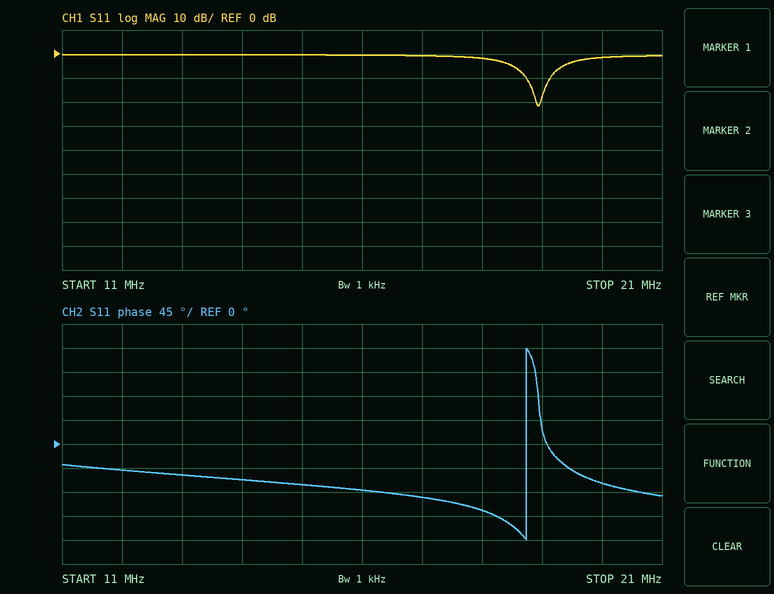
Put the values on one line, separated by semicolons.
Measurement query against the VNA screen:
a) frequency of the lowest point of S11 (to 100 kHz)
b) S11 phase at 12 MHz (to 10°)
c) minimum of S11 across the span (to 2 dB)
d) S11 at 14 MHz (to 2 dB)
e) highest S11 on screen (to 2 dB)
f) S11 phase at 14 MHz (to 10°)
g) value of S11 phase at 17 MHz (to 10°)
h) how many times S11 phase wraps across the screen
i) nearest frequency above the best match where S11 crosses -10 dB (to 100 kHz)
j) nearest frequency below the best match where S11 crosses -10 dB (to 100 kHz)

18.9 MHz; -50°; -22 dB; 0 dB; 0 dB; -70°; -100°; 1; 19.1 MHz; 18.7 MHz
